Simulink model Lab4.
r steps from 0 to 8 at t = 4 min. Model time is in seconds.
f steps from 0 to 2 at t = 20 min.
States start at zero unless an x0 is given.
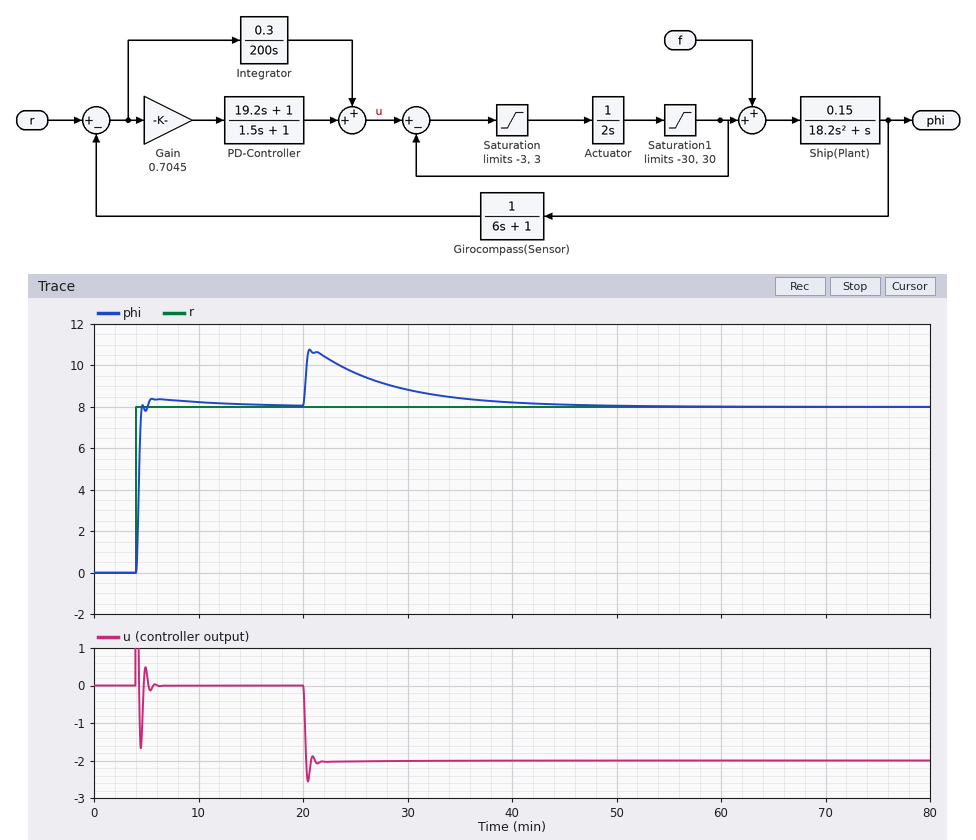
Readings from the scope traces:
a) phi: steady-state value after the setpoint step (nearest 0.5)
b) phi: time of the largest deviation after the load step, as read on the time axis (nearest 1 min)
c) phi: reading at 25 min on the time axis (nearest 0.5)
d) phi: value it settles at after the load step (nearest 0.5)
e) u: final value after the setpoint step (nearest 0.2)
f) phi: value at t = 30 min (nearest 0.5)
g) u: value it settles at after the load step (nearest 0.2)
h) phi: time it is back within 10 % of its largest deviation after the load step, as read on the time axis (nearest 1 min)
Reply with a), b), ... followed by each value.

a) 8.0
b) 21 min
c) 9.5
d) 8.0
e) 0.0
f) 9.0
g) -2.0
h) 38 min
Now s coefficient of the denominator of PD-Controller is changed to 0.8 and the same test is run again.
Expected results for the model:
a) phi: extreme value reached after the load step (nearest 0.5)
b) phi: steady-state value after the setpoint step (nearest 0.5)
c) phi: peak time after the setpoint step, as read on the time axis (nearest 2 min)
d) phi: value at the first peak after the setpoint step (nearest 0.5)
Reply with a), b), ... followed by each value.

a) 10.5
b) 8.0
c) 6 min
d) 8.5
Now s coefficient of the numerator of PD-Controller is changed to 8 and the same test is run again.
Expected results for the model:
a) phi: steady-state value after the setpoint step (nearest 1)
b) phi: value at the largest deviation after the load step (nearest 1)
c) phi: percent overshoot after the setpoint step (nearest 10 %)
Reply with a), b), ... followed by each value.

a) 8
b) 12
c) 40 %
